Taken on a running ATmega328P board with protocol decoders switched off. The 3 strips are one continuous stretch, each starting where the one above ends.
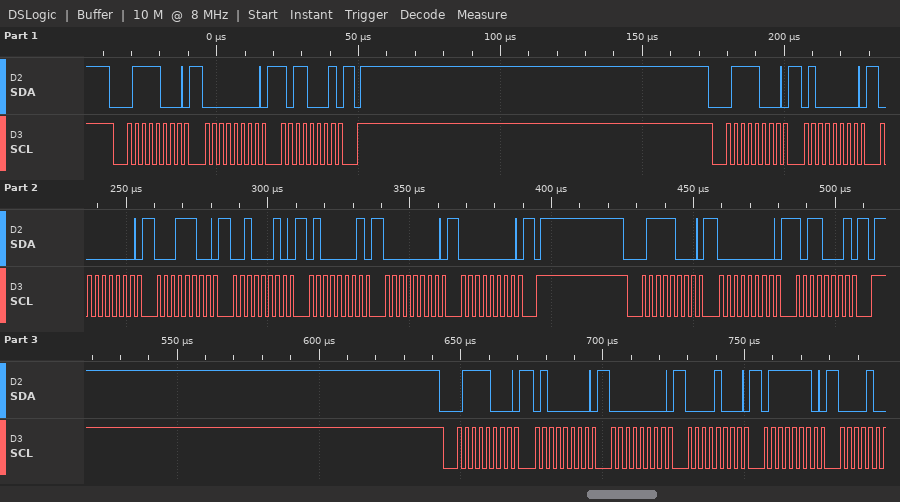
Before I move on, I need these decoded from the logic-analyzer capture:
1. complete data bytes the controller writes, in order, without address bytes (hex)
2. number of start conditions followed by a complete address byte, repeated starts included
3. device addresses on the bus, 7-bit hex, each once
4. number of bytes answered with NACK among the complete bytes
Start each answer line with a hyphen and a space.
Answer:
- 00 B1 40 00 1C 22 41 00 00 00 B1 40 00 08 7E
- 4
- 0x3C
- 0
